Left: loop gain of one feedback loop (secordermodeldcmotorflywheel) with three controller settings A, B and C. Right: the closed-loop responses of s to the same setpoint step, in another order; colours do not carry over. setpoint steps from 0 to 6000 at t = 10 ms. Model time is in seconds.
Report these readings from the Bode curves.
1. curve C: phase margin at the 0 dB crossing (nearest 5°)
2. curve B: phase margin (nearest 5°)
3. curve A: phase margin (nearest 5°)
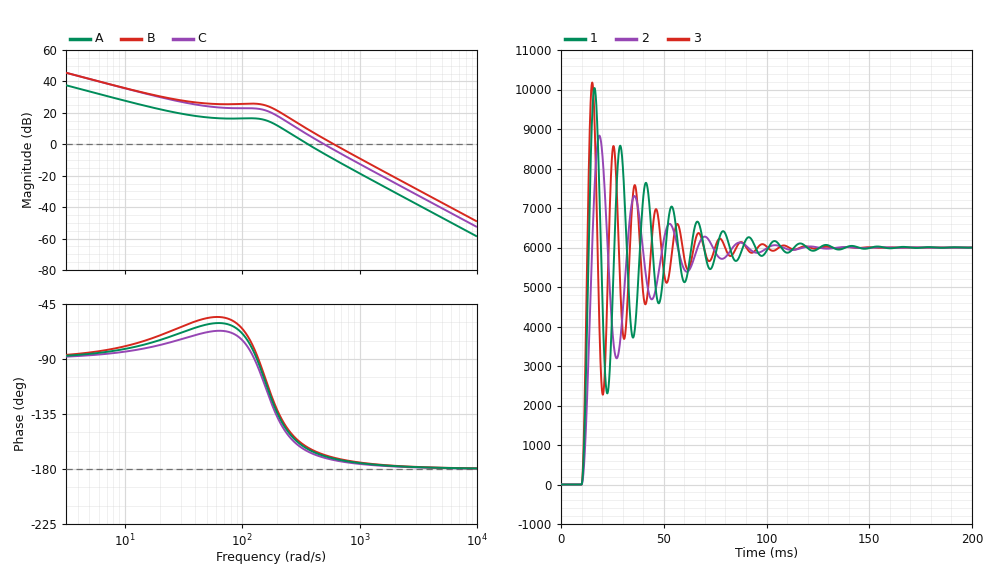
10°
10°
15°
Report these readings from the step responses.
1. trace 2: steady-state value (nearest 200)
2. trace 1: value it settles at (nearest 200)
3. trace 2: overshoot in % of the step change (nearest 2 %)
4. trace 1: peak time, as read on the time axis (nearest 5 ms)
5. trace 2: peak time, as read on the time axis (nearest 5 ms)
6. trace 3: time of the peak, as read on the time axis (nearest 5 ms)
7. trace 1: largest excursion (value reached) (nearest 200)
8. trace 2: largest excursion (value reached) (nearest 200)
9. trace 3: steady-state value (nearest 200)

6000
6000
48 %
15 ms
20 ms
15 ms
10000
8800
6000
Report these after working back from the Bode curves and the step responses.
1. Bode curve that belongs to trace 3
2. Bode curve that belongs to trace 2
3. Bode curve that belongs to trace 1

B
A
C
